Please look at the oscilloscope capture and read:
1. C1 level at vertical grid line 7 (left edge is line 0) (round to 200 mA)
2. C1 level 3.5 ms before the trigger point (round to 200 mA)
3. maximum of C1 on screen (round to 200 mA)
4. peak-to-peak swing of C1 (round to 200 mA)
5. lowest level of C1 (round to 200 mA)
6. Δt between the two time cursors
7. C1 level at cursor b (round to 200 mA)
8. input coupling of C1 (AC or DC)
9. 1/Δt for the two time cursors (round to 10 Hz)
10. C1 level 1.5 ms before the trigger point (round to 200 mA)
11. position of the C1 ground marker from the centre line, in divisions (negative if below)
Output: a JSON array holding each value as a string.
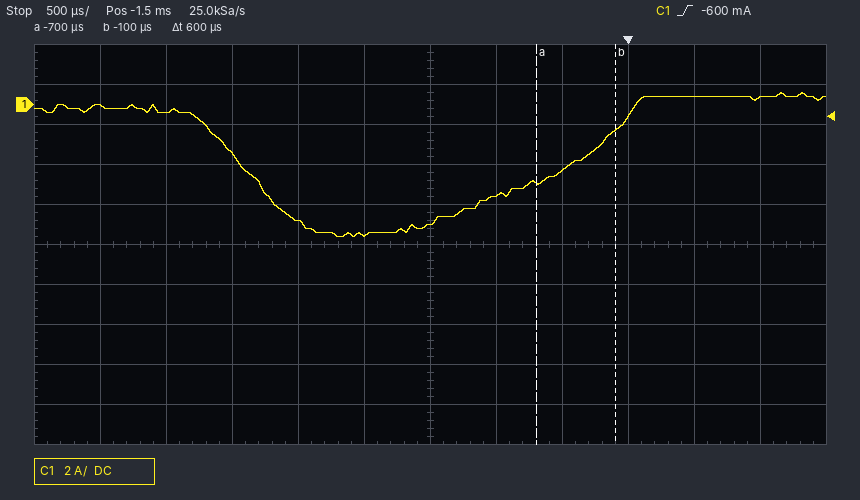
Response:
["-4.6 A", "-400 mA", "600 mA", "7.2 A", "-6.6 A", "600 µs", "-1.2 A", "DC", "1.67 kHz", "-6.0 A", "+3.5 div"]
